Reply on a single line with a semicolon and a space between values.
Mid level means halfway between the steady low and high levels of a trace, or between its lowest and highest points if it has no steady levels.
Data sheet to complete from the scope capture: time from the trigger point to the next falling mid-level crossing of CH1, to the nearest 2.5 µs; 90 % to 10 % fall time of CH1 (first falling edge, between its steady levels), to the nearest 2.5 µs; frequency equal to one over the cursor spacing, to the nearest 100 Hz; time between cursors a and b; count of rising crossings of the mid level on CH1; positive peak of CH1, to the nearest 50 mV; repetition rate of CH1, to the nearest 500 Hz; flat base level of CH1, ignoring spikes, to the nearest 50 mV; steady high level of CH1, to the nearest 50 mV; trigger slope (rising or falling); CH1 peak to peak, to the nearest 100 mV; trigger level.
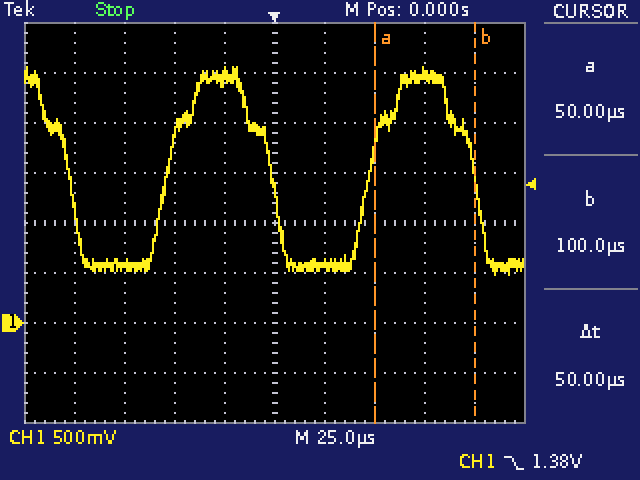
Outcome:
100.0 µs; 20.0 µs; 20.0 kHz; 50 µs; 2; 2.55 V; 10.0 kHz; 550 mV; 2.45 V; falling; 2.10 V; 1.38 V
